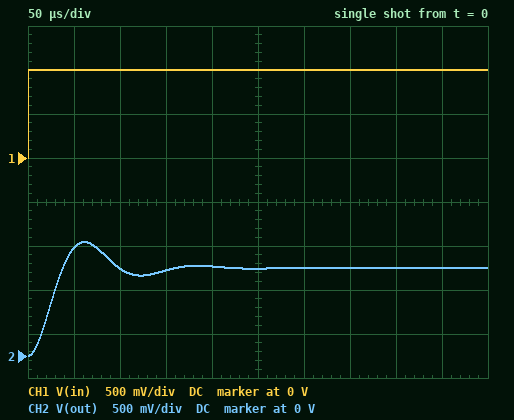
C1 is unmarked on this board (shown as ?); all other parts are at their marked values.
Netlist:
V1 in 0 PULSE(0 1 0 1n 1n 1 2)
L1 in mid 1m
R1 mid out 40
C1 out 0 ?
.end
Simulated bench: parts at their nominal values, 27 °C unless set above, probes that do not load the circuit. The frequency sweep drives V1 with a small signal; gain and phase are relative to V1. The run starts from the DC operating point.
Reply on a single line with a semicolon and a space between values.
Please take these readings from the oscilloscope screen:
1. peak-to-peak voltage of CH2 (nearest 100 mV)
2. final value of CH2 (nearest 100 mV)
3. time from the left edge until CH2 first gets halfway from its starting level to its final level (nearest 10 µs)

1.3 V; 1.0 V; 20 µs
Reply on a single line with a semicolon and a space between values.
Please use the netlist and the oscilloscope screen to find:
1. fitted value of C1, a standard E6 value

330 nF
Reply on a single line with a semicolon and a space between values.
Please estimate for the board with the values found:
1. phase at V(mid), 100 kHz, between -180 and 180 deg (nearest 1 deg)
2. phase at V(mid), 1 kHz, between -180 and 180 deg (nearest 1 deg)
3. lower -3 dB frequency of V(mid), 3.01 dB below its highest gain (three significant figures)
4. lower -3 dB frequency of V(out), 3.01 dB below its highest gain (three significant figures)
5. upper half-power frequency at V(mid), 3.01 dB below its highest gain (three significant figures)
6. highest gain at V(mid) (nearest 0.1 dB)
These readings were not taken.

-93 deg; 0 deg; 4.11 kHz; 2.13 kHz; 11.1 kHz; 4.9 dB
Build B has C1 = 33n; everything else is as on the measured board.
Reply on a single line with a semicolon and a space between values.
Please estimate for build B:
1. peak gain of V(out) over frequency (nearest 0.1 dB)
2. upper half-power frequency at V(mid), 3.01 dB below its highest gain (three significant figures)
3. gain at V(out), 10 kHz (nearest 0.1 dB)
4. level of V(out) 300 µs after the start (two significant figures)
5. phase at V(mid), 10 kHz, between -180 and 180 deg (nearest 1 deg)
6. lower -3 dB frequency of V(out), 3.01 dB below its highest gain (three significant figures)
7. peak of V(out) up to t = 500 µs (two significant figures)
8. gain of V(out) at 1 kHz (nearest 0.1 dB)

12.8 dB; 30.4 kHz; 1.2 dB; 1.0 V; -1 deg; 23.9 kHz; 1.7 V; 0 dB
